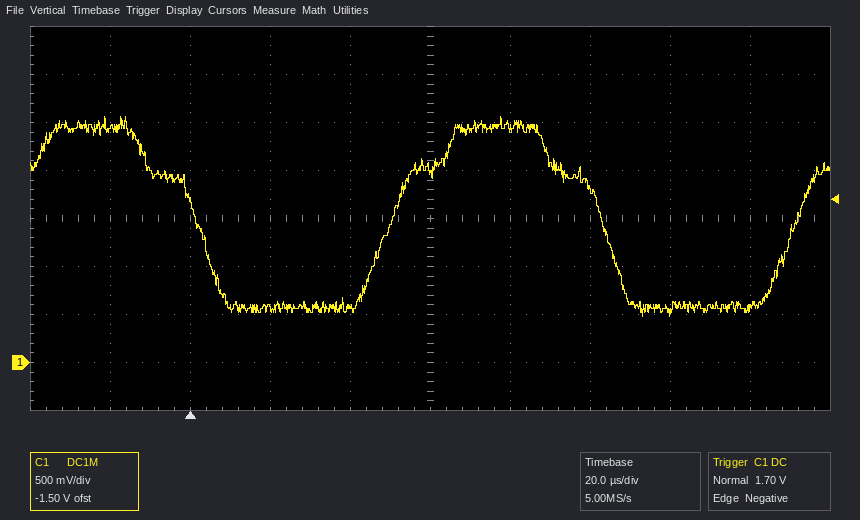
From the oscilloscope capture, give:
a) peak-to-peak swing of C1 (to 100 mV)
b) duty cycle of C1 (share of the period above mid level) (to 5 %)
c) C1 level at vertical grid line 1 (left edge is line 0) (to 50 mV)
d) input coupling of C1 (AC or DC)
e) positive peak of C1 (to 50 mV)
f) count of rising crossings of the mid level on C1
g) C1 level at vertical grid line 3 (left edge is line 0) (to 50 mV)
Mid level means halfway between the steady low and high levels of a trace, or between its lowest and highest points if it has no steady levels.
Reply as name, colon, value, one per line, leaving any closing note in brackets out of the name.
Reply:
peak-to-peak swing of C1: 2.10 V
duty cycle of C1 (share of the period above mid level): 50 %
C1 level at vertical grid line 1 (left edge is line 0): 2.45 V
input coupling of C1: DC
positive peak of C1: 2.55 V
count of rising crossings of the mid level on C1: 2
C1 level at vertical grid line 3 (left edge is line 0): 550 mV
